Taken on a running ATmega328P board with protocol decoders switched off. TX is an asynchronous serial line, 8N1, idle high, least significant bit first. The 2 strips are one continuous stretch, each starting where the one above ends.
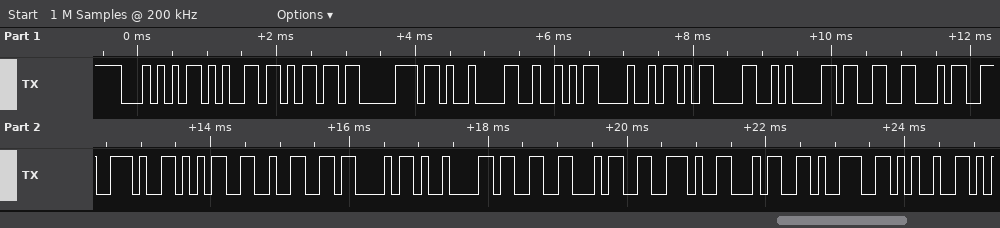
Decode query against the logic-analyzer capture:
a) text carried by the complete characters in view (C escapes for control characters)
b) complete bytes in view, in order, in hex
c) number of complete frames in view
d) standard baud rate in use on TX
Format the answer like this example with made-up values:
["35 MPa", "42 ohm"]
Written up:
["\"Temp\\tRH\\r\\n34.52C\\t34.49%\"", "54 65 6D 70 09 52 48 0D 0A 33 34 2E 35 32 43 09 33 34 2E 34 39 25", "22", "9600 baud"]
